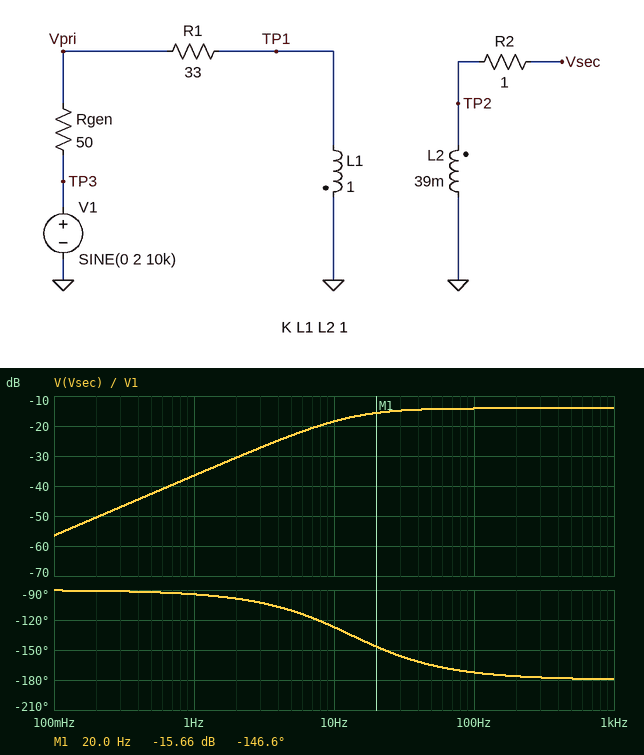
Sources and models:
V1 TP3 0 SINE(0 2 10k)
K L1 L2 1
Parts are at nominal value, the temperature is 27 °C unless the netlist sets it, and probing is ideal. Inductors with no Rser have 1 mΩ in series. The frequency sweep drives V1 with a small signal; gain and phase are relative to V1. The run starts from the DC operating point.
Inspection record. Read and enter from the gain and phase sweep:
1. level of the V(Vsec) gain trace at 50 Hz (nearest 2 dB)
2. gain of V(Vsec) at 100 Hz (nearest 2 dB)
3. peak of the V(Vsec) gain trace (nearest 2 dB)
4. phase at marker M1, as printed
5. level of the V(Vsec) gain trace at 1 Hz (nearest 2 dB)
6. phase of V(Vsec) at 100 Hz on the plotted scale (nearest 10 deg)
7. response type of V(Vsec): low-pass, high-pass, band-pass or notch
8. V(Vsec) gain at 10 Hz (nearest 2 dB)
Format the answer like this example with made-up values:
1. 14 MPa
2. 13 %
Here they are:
1. -14 dB
2. -14 dB
3. -14 dB
4. -146.6 deg
5. -36 dB
6. -170 deg
7. high-pass
8. -18 dB
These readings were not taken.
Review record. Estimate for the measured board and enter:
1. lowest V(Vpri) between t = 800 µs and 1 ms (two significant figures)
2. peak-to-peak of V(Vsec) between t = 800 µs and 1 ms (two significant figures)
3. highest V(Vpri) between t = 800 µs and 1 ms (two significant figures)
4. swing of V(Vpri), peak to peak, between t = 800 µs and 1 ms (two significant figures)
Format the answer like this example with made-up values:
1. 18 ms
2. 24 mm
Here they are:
1. -2.0 V
2. 790 mV
3. 2.0 V
4. 4.0 V
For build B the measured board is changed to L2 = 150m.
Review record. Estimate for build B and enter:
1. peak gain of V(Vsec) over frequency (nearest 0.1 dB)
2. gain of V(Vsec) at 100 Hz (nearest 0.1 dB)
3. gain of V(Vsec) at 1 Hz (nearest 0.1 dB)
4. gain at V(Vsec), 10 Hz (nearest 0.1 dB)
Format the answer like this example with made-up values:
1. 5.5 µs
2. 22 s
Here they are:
1. -8.2 dB
2. -8.3 dB
3. -30.7 dB
4. -12.6 dB
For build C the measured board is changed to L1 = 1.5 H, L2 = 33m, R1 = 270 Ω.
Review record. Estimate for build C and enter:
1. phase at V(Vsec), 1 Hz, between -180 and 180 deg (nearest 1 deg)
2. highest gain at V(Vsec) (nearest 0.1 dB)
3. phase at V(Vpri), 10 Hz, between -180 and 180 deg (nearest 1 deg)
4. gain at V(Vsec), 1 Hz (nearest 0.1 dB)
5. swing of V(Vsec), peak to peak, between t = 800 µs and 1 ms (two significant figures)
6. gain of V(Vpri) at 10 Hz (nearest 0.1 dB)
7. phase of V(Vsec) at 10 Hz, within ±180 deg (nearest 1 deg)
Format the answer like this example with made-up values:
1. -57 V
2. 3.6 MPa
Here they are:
1. -92 deg
2. -16.6 dB
3. 3 deg
4. -47.2 dB
5. 590 mV
6. -1.3 dB
7. -106 deg
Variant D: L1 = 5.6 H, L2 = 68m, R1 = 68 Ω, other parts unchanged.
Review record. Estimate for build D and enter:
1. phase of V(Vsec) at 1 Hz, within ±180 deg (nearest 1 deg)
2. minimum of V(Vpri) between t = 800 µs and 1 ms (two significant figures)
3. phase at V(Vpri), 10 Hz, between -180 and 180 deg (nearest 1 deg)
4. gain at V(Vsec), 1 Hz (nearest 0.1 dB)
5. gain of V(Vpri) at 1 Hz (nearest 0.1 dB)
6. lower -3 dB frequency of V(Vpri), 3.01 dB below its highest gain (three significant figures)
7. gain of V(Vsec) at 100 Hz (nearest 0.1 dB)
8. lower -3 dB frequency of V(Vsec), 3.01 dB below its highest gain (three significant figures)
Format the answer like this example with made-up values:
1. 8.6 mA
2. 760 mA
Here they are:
1. -107 deg
2. -2.0 V
3. 8 deg
4. -30.0 dB
5. -4.1 dB
6. 1.94 Hz
7. -19.2 dB
8. 3.35 Hz
